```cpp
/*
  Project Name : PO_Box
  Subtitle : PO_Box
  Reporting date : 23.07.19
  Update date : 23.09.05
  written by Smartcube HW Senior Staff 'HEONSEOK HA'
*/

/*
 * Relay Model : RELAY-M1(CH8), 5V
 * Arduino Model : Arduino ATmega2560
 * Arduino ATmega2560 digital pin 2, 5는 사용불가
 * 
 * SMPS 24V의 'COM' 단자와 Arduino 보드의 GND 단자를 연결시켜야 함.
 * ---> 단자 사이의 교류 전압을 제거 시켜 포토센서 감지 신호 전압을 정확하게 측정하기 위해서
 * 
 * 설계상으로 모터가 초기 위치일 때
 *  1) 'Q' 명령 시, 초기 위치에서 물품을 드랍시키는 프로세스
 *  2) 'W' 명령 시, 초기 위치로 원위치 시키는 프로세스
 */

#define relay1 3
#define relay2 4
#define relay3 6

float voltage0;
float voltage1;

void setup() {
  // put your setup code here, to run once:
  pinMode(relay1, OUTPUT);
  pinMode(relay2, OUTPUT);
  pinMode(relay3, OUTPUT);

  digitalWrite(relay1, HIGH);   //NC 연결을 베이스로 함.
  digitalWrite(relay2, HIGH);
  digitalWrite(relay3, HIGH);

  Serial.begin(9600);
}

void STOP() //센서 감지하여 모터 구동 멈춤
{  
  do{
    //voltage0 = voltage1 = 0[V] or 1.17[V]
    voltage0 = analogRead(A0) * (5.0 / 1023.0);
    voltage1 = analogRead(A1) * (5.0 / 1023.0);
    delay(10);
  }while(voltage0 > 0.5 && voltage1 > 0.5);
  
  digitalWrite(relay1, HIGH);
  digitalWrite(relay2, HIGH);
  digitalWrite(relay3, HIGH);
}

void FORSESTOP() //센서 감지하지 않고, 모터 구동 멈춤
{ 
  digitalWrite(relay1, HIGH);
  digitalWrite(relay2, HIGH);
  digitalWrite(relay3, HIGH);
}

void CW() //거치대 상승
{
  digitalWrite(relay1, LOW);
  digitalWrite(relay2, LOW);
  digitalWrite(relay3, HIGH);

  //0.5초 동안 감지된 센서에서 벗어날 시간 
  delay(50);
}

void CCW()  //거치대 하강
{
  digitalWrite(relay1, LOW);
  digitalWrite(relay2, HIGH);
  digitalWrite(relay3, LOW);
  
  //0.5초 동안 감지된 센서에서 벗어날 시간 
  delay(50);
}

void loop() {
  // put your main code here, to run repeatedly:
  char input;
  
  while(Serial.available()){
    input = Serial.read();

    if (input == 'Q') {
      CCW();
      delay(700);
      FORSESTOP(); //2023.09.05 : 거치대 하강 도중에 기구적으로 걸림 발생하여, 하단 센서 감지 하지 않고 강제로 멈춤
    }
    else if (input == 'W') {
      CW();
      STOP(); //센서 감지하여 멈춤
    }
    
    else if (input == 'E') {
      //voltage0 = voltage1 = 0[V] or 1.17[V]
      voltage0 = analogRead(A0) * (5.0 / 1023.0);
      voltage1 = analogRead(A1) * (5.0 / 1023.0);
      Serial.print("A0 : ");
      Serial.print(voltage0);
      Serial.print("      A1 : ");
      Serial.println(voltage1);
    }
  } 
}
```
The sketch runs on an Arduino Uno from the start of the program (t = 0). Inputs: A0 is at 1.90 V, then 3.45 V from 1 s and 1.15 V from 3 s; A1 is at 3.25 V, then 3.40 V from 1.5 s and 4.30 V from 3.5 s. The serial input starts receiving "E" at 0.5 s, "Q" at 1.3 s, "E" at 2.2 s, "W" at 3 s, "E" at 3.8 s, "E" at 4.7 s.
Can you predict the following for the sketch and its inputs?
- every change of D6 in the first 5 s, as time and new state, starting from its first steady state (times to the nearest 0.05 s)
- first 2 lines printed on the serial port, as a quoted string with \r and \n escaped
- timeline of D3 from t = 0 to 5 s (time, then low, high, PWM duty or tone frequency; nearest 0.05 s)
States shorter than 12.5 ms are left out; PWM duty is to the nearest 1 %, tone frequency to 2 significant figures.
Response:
0 s high; 1.3 s low; 2.05 s high
"A0 : 1.90      A1 : 3.25\r\nA0 : 3.45      A1 : 3.40\r\n"
0 s high; 1.3 s low; 2.05 s high; 3 s low
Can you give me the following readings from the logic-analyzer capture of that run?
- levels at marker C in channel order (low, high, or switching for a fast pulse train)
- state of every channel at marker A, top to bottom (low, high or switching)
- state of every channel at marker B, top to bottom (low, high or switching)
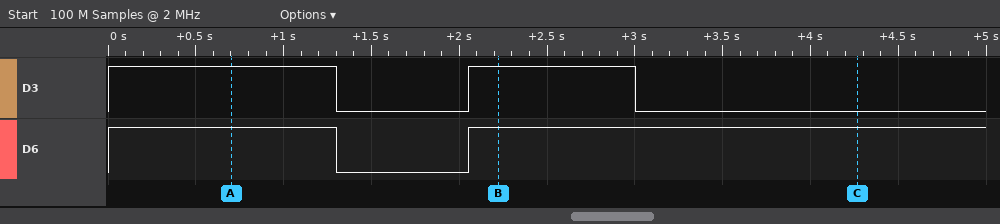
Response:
D3 low, D6 high
D3 high, D6 high
D3 high, D6 high
